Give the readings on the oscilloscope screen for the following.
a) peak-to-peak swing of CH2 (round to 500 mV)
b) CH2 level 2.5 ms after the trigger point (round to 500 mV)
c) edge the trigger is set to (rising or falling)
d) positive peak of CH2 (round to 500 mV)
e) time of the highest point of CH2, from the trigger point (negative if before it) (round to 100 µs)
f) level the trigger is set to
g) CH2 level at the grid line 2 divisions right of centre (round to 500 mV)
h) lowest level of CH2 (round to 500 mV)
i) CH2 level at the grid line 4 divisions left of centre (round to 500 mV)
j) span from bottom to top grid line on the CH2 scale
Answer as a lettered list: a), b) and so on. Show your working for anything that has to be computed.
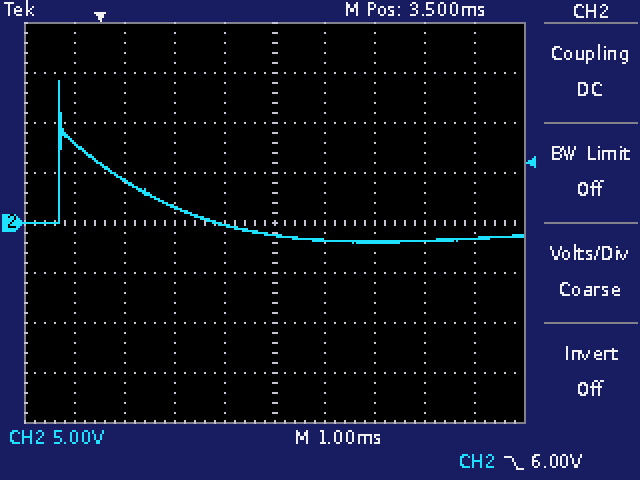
a) 14.0 V − (-2.0 V) = 16.0 V
b) 0.0 V
c) falling
d) 14.0 V
e) -800 µs
f) 6.00 V
g) -2.0 V
h) -2.0 V
i) 8.0 V
j) 40 V
